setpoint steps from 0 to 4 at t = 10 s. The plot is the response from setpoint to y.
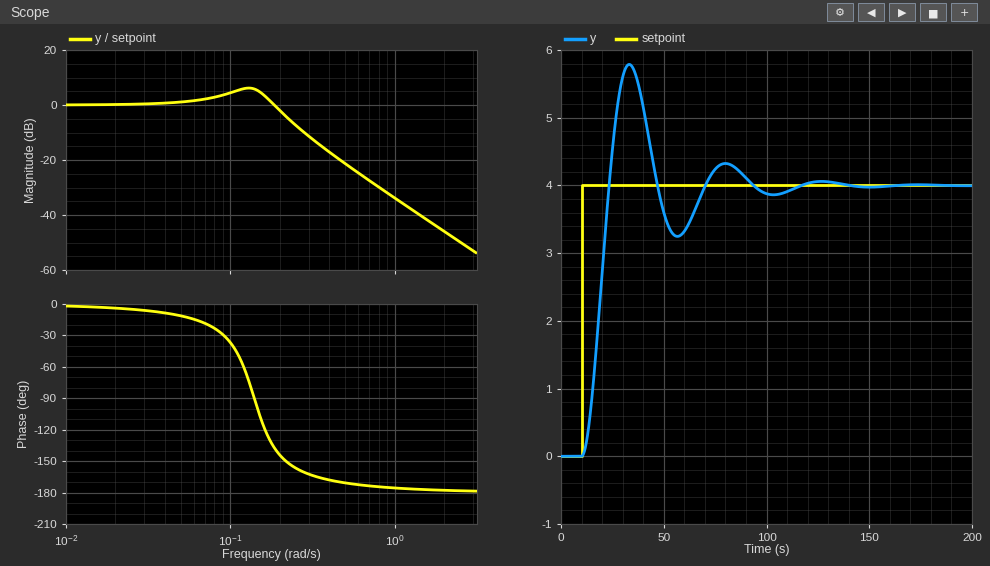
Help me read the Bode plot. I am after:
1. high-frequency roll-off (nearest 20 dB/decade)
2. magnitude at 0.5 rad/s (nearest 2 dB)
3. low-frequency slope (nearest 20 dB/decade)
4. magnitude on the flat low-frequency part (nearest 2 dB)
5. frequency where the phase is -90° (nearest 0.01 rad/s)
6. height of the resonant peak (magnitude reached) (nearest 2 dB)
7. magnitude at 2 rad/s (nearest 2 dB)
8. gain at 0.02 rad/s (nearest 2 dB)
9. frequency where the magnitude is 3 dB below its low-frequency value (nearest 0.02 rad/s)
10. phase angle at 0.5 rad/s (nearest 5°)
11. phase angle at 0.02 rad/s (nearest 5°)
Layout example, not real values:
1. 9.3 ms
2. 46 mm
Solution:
1. -40 dB/decade
2. -22 dB
3. 0 dB/decade
4. 0 dB
5. 0.14 rad/s
6. 6 dB
7. -46 dB
8. 0 dB
9. 0.20 rad/s
10. -170°
11. -5°
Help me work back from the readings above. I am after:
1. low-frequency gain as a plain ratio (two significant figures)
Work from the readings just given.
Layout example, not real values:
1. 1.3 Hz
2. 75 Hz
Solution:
1. 1.0
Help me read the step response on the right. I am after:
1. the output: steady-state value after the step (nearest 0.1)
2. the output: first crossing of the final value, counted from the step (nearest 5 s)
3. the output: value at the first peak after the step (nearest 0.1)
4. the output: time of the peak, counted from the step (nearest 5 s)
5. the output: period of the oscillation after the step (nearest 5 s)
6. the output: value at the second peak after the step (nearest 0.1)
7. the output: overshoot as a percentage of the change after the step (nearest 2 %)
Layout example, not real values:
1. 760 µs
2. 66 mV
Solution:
1. 4.0
2. 15 s
3. 5.8
4. 25 s
5. 45 s
6. 4.3
7. 44 %
